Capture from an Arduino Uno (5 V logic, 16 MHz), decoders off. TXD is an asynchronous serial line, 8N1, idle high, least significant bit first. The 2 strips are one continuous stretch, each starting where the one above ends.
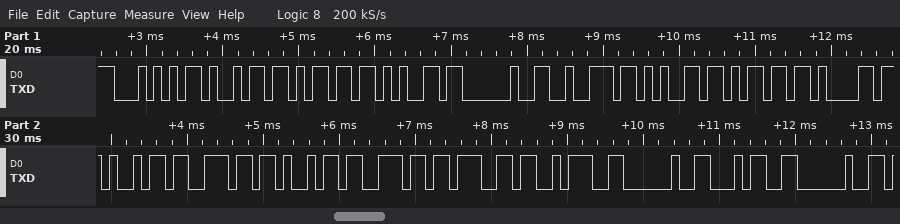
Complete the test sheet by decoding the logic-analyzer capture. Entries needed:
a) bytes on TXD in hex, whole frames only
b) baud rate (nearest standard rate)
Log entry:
54 69 6D 65 20 72 65 6D 61 69 6E 69 6E 67 3A 20 34 20
9600 baud
